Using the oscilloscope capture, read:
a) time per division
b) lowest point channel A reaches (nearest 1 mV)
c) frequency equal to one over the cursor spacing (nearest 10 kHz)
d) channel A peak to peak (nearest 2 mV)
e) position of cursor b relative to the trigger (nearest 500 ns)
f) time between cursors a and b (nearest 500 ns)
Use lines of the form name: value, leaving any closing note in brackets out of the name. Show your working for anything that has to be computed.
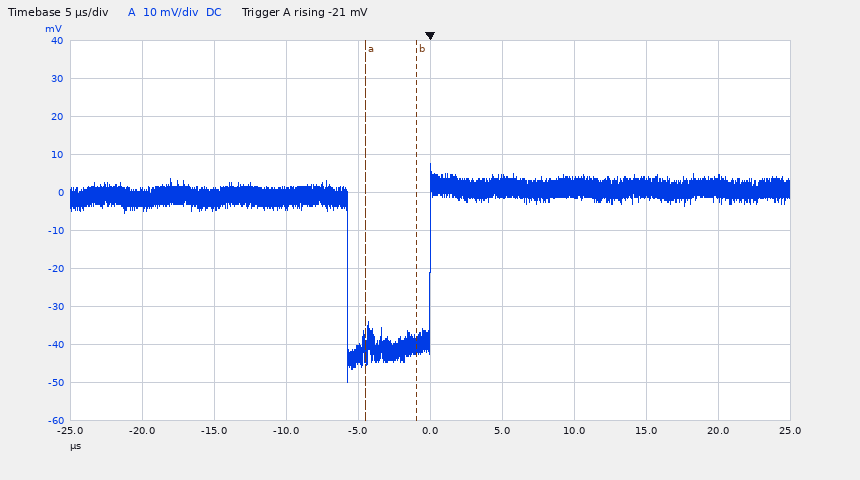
time per division: 5 µs
lowest point channel A reaches: -50 mV
frequency equal to one over the cursor spacing: 1 / 3.5 µs ≈ 290 kHz
channel A peak to peak: 58 mV
position of cursor b relative to the trigger: -1.0 µs
time between cursors a and b: 3.5 µs
